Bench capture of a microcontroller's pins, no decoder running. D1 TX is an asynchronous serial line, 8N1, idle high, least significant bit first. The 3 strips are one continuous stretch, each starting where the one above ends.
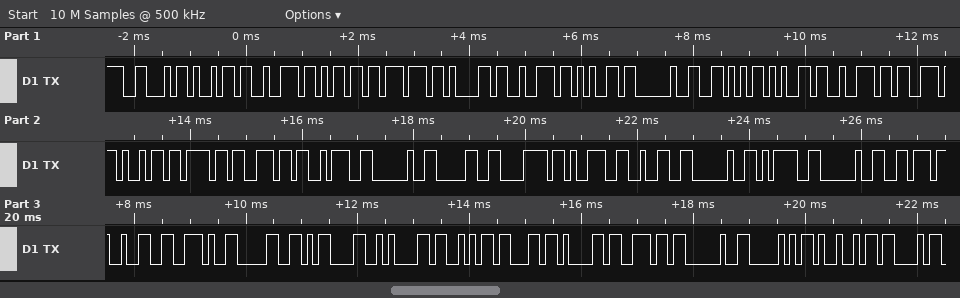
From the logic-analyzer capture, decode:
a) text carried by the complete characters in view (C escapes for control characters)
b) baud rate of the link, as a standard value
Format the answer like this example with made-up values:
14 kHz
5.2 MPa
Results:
"Firmware Version: 0x92 = v2.0\r\nScan PIC"
9600 baud
